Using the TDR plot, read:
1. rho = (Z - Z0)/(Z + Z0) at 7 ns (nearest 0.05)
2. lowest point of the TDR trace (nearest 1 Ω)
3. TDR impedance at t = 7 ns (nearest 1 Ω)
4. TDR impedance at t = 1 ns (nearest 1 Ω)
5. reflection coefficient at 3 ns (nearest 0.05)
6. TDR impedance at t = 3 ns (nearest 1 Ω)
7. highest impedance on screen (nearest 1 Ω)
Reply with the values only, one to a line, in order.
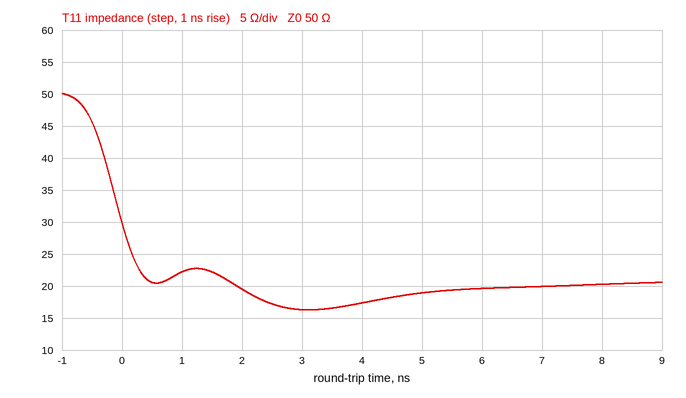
-0.45
16 Ω
20 Ω
22 Ω
-0.50
16 Ω
50 Ω
